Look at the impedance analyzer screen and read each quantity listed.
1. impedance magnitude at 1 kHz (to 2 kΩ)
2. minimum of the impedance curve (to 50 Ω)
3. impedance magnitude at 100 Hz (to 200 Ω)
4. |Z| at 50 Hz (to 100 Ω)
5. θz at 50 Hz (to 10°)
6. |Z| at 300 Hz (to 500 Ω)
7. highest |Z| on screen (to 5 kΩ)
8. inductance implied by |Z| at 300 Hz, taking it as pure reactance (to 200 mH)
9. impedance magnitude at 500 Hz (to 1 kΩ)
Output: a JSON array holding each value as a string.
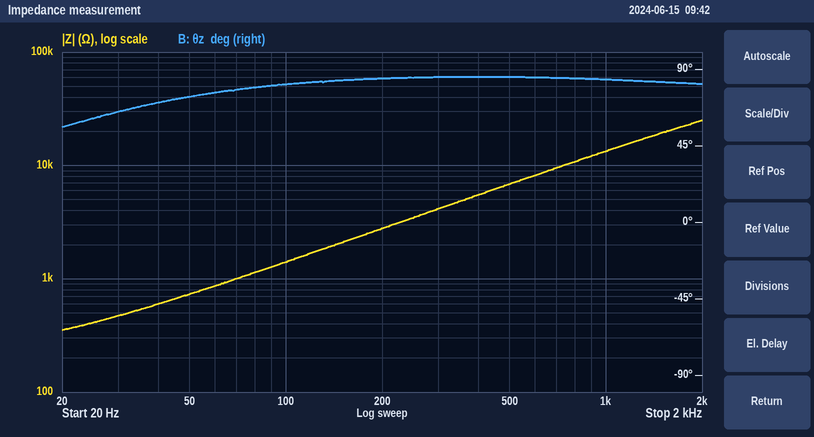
["14 kΩ", "350 Ω", "1.4 kΩ", "700 Ω", "70°", "4.0 kΩ", "25 kΩ", "2.2 H", "7 kΩ"]
